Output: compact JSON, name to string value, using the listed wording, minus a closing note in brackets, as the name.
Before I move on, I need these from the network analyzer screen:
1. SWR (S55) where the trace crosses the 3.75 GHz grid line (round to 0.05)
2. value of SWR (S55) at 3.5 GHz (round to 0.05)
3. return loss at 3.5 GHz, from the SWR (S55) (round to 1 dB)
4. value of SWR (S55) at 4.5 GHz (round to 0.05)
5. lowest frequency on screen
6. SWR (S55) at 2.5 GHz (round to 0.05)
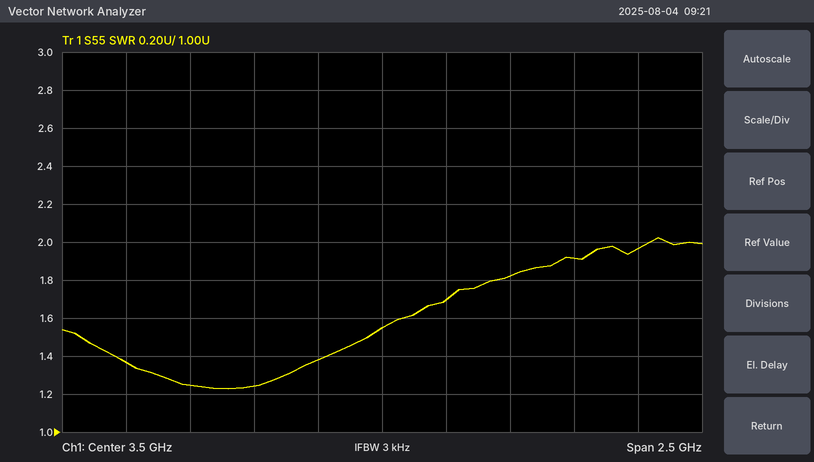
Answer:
{"SWR (S55) where the trace crosses the 3.75 GHz grid line": "1.70", "value of SWR (S55) at 3.5 GHz": "1.55", "return loss at 3.5 GHz, from the SWR (S55)": "13 dB", "value of SWR (S55) at 4.5 GHz": "1.95", "lowest frequency on screen": "2.25 GHz", "SWR (S55) at 2.5 GHz": "1.35"}
